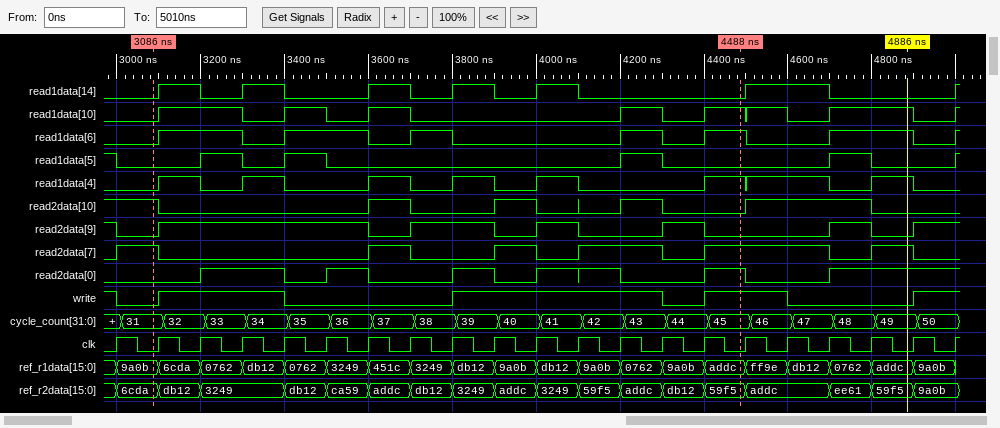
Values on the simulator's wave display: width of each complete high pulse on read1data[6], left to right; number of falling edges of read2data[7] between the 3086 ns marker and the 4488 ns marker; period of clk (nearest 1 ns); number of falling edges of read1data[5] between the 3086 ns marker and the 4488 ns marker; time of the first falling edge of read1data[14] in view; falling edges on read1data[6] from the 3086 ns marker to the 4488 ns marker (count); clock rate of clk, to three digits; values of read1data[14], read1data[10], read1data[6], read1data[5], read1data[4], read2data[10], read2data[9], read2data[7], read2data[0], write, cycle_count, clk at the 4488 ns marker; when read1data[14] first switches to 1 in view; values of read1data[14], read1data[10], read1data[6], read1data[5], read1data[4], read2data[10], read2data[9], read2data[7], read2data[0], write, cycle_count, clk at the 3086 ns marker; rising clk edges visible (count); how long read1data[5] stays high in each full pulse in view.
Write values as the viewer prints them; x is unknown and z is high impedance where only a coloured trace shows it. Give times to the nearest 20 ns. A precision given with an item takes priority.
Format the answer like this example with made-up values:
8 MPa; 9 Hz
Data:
200 ns, 200 ns, 100 ns, 100 ns, 100 ns, 200 ns; 4; 100 ns; 3; 3200 ns; 4; 10.0 MHz; read1data[14]=0, read1data[10]=1, read1data[6]=1, read1data[5]=0, read1data[4]=1, read2data[10]=0, read2data[9]=0, read2data[7]=1, read2data[0]=1, write=1, cycle_count=45, clk=0; 3100 ns; read1data[14]=0, read1data[10]=0, read1data[6]=0, read1data[5]=0, read1data[4]=0, read2data[10]=1, read2data[9]=0, read2data[7]=1, read2data[0]=0, write=0, cycle_count=31, clk=0; 21; 100 ns, 100 ns, 100 ns, 100 ns
